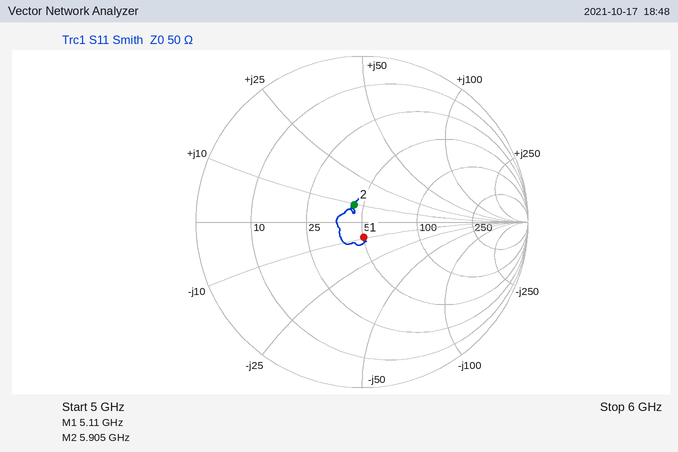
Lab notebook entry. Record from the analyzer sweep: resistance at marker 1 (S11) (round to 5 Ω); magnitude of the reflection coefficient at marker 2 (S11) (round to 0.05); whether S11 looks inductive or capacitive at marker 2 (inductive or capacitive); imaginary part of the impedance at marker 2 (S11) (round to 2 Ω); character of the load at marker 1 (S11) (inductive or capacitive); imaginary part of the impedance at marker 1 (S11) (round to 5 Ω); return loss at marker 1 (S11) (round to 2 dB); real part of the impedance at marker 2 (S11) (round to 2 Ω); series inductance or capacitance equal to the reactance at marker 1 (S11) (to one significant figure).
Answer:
50 Ω
0.10
inductive
+10 Ω
capacitive
-10 Ω
20 dB
44 Ω
3 pF
